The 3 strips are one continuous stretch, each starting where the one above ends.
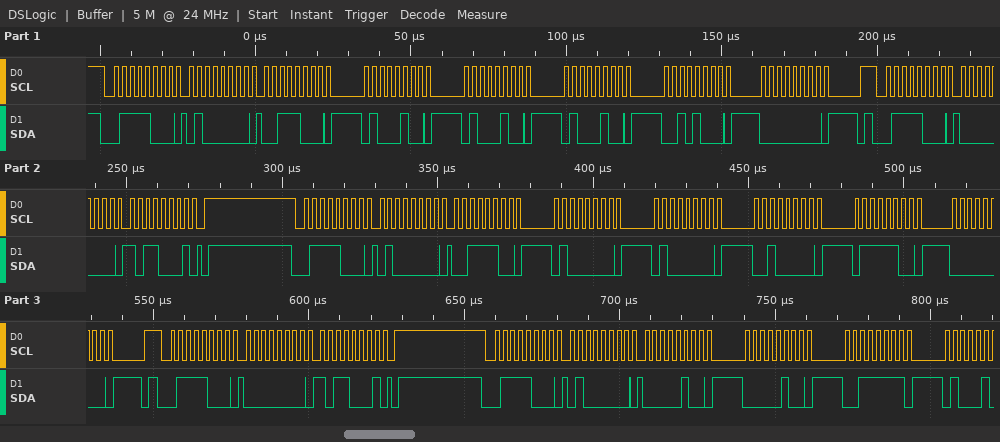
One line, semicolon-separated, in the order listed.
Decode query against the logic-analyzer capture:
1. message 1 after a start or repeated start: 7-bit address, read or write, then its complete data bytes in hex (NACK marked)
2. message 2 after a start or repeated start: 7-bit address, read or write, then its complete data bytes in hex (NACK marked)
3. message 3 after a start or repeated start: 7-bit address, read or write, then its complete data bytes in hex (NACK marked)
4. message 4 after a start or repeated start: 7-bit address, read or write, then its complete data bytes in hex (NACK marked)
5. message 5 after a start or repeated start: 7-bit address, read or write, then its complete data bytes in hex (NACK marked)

0x3C write: 40 38 44 44 44 28 00; 0x3C write: 00 B1; 0x3C write: 40 3C 40 40 20 7C 00; 0x3C write: 00 B1; 0x3C write: 40 04 04 3F
